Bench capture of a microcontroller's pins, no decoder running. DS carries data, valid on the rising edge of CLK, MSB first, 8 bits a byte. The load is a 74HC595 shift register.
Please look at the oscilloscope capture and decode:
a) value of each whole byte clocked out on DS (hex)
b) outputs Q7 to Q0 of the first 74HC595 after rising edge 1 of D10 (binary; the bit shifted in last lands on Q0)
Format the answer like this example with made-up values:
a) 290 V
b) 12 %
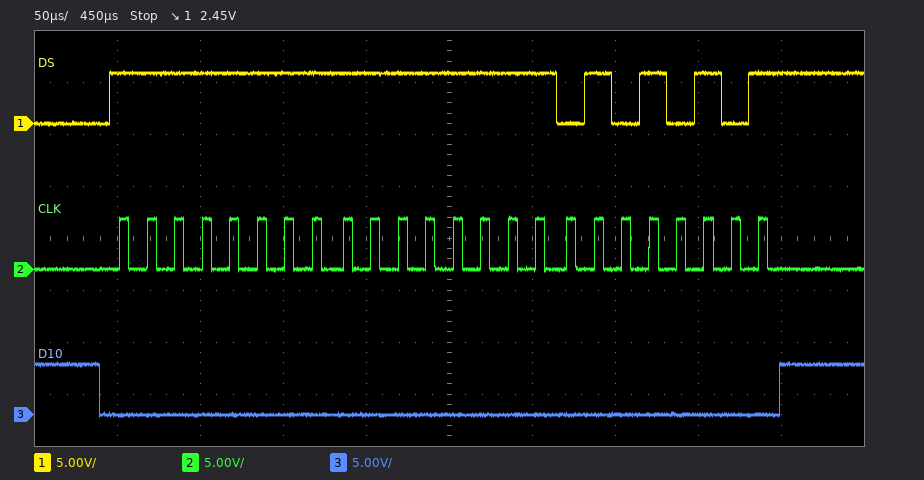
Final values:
a) FF FF 55
b) 01010101
